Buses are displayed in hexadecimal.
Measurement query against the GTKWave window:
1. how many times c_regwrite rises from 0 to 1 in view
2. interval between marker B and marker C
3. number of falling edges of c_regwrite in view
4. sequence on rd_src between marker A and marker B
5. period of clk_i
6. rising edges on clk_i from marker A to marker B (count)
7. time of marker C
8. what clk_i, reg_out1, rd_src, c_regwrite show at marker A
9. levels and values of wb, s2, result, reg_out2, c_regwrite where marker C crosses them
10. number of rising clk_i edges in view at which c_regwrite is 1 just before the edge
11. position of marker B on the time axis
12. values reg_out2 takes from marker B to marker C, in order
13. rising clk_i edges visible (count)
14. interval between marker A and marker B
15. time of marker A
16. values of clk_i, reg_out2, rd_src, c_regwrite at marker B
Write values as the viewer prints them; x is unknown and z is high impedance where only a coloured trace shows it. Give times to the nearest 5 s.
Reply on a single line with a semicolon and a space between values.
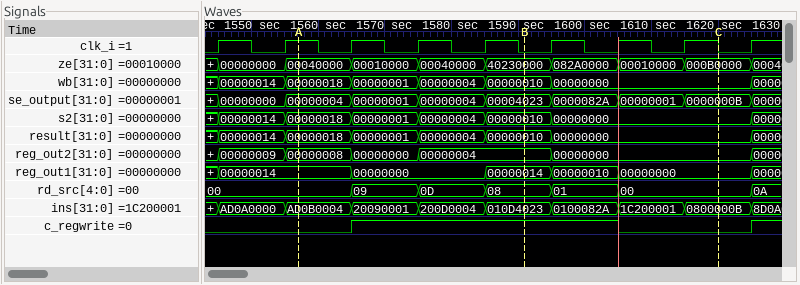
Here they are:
2; 30 s; 1; 00, 09, 0D, 08; 10 s; 3; 1620 s; clk_i=1, reg_out1=00000014, rd_src=00, c_regwrite=0; wb=00000000, s2=00000000, result=00000000, reg_out2=00000000, c_regwrite=0; 4; 1590 s; 00000004, 00000000; 9; 35 s; 1555 s; clk_i=0, reg_out2=00000004, rd_src=08, c_regwrite=1
